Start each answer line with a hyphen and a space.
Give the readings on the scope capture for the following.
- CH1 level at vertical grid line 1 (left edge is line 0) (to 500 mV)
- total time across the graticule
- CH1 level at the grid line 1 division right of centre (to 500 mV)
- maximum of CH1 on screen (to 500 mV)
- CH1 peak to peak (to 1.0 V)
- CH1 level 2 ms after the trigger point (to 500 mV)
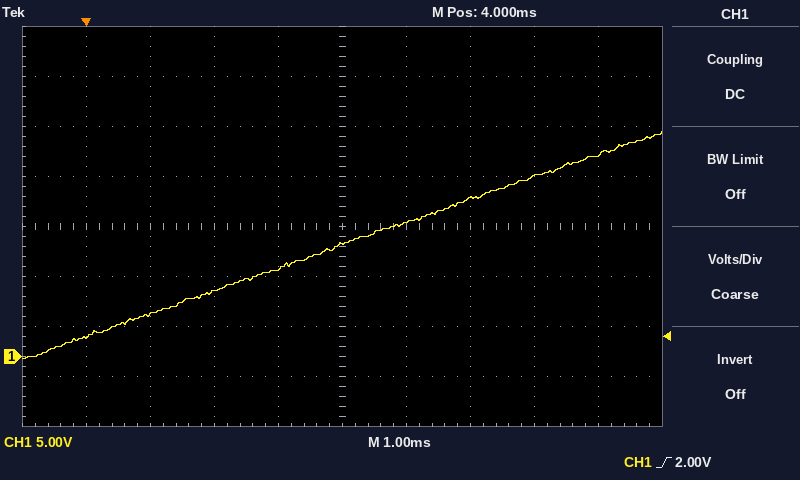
- 2.0 V
- 10 ms
- 13.5 V
- 22.5 V
- 23.0 V
- 6.5 V
